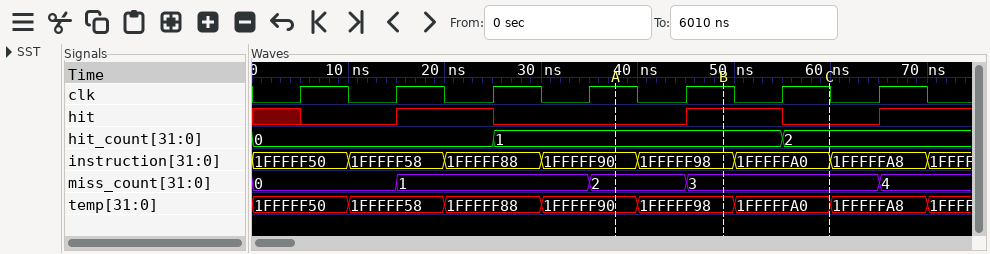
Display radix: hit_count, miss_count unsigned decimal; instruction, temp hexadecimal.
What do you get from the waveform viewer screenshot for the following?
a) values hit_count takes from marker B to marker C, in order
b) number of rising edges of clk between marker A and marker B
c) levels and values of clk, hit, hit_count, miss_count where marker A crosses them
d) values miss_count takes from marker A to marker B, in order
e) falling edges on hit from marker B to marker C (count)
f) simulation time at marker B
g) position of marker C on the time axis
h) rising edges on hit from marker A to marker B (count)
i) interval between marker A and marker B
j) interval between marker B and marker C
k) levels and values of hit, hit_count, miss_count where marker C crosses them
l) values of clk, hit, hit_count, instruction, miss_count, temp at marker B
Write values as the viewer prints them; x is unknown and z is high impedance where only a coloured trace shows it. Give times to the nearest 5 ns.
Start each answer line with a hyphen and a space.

- 1, 2
- 1
- clk=1, hit=0, hit_count=1, miss_count=2
- 2, 3
- 1
- 50 ns
- 60 ns
- 1
- 10 ns
- 10 ns
- hit=0, hit_count=2, miss_count=3
- clk=1, hit=1, hit_count=1, instruction=1FFFFF98, miss_count=3, temp=1FFFFF98
